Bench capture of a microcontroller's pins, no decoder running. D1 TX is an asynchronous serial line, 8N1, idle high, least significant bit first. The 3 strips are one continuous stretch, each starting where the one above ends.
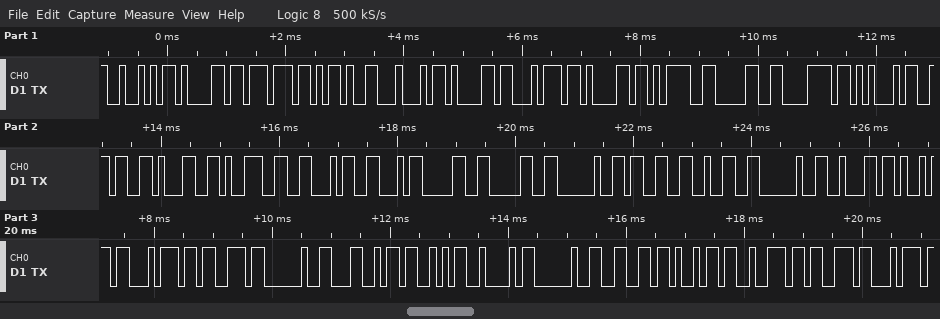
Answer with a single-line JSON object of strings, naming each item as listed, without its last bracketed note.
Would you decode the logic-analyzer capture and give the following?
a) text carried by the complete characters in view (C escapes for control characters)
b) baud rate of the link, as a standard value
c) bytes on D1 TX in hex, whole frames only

{"text carried by the complete characters in view": "\"Raw-Data=0xE619FF00 32 bits LSB first\"", "baud rate of the link, as a standard value": "9600 baud", "bytes on D1 TX in hex, whole frames only": "52 61 77 2D 44 61 74 61 3D 30 78 45 36 31 39 46 46 30 30 20 33 32 20 62 69 74 73 20 4C 53 42 20 66 69 72 73 74"}
